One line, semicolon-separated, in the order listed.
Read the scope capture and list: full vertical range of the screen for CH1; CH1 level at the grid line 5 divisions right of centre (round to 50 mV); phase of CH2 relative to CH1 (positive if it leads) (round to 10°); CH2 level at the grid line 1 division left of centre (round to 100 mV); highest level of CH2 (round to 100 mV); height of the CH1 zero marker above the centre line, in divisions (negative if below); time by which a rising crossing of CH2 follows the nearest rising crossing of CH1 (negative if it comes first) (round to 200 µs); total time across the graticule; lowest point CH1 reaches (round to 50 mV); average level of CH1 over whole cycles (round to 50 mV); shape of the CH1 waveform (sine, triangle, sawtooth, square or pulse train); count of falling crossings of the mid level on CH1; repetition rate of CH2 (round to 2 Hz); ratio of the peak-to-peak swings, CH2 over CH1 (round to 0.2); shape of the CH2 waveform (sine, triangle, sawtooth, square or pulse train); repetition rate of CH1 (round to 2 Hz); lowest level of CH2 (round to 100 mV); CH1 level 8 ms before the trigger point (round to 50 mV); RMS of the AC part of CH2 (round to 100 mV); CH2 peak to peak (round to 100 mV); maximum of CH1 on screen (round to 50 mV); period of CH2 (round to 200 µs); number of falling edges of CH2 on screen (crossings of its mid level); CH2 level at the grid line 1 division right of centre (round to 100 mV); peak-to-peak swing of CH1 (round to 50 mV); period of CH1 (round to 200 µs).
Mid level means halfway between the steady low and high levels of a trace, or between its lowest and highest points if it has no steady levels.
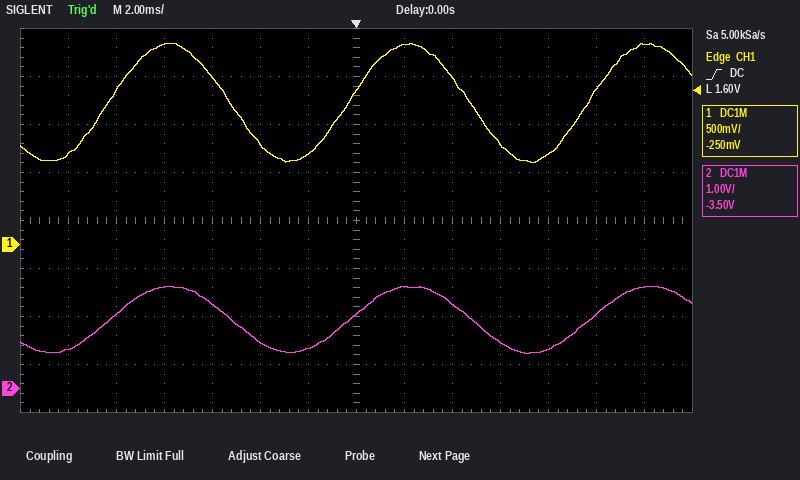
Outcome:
4 V; 1.60 V; 0°; 800 mV; 2.1 V; -0.5 div; 0.0 ms; 28 ms; 850 mV; 1.50 V; sine; 2; 100 Hz; 1.2; sine; 100 Hz; 700 mV; 2.10 V; 500 mV; 1.4 V; 2.10 V; 10.0 ms; 2; 2.1 V; 1.25 V; 10.0 ms
